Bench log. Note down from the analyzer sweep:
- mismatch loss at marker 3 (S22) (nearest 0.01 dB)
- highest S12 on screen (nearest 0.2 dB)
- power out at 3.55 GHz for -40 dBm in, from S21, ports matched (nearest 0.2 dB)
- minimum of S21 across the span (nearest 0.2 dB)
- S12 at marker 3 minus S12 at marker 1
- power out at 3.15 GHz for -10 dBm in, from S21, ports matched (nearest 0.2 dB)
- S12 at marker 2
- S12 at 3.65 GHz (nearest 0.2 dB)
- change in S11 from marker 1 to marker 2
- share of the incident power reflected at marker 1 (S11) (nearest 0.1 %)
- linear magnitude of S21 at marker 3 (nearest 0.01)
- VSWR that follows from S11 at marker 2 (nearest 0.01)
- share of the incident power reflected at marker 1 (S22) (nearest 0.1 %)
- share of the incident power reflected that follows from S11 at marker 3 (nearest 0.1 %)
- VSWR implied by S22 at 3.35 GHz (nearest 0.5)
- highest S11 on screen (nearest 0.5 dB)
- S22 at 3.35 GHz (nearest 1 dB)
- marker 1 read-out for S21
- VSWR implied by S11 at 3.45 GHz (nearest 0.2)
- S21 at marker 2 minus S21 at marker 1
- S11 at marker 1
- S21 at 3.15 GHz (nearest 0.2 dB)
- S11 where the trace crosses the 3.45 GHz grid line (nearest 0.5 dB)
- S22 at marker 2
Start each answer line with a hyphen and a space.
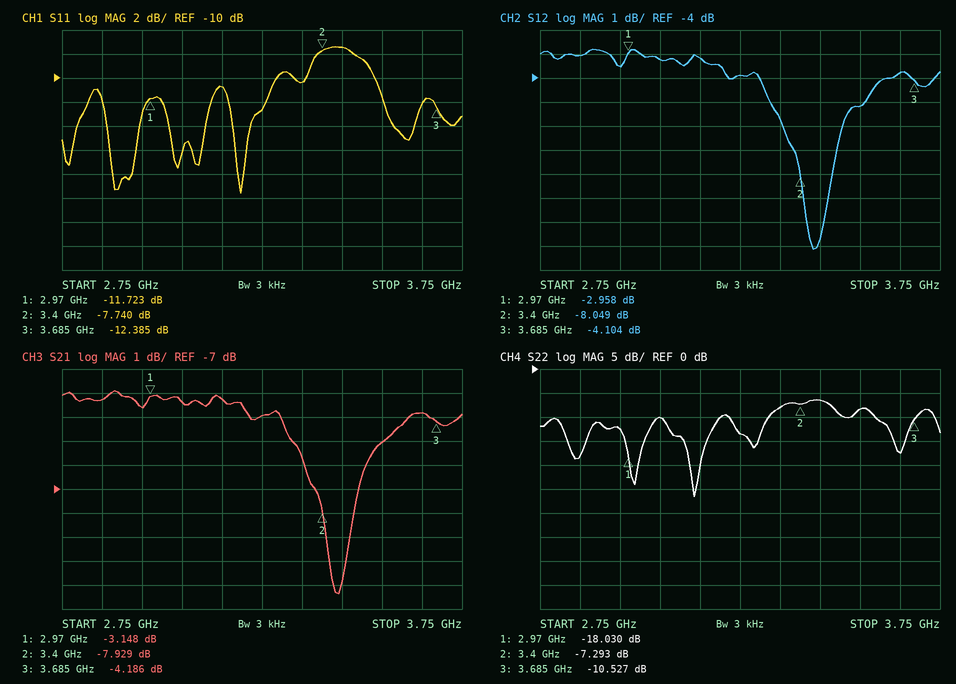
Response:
- 0.40 dB
- -2.8 dB
- -45.0 dBm
- -11.4 dB
- -1.146 dB
- -13.2 dBm
- -8.049 dB
- -3.8 dB
- 3.983 dB
- 6.7 %
- 0.62
- 2.39
- 1.6 %
- 5.8 %
- 2.5
- -7.5 dB
- -8 dB
- -3.148 dB
- 2.4
- -4.781 dB
- -11.723 dB
- -3.2 dB
- -7.5 dB
- -7.293 dB
